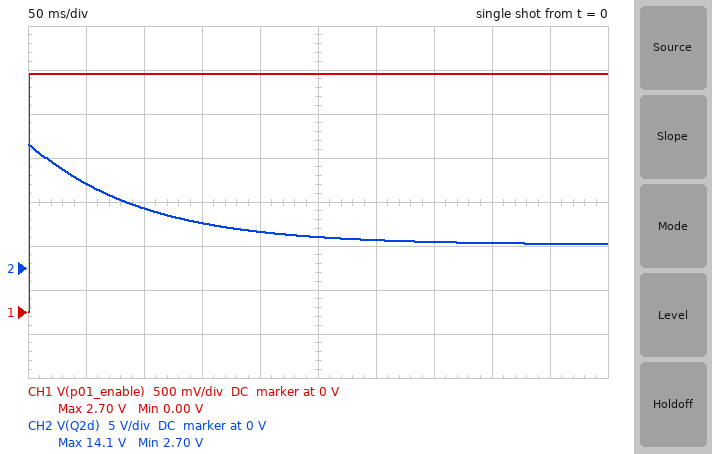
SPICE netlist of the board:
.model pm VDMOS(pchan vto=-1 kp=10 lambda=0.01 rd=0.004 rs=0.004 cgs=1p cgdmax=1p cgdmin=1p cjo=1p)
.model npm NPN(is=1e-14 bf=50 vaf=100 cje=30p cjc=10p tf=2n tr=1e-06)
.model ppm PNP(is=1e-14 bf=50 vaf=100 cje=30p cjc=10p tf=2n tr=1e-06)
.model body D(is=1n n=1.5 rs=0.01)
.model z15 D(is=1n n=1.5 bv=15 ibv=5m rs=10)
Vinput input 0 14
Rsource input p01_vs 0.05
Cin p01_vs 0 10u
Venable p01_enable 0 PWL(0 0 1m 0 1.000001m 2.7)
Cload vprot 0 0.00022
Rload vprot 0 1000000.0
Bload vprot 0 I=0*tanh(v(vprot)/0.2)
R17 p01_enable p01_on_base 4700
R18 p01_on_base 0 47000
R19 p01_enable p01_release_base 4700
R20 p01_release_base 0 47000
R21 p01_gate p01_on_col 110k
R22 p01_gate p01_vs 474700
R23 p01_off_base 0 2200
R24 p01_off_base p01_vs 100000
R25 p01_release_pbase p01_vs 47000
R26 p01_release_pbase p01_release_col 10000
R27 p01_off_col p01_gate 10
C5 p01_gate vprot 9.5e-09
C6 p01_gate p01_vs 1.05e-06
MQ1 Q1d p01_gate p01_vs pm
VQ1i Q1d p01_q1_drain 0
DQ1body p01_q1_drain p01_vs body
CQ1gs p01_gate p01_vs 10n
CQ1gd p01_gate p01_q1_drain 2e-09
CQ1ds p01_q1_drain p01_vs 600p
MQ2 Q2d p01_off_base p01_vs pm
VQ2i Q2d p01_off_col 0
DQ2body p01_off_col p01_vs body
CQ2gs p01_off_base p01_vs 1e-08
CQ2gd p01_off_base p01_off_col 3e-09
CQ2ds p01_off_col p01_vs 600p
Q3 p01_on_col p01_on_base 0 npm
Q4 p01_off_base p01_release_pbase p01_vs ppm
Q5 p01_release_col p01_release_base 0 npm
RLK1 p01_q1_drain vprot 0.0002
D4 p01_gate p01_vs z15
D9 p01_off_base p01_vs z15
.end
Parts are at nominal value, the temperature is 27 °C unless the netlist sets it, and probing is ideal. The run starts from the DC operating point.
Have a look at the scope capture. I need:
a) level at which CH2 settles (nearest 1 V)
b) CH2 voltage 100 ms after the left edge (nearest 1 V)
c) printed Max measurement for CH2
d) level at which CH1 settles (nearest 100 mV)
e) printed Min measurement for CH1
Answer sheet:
3 V
7 V
14.1 V
2.7 V
0.00 V
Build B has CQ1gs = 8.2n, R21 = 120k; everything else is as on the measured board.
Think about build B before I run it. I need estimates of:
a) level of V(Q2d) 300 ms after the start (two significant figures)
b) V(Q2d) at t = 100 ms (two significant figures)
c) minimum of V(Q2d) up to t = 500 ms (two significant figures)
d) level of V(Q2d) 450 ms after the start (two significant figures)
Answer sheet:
3.5 V
7.2 V
2.9 V
3.0 V
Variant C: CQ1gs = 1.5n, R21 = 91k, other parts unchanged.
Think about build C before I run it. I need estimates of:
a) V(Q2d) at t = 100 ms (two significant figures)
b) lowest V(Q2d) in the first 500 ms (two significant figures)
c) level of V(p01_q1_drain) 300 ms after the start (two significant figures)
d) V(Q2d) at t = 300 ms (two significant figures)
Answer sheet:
5.8 V
2.3 V
14 V
2.6 V
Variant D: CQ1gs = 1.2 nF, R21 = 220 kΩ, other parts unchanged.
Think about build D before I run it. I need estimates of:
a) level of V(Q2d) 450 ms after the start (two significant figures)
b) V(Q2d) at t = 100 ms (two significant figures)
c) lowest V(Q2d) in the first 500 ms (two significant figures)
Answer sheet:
5.0 V
9.7 V
4.9 V
